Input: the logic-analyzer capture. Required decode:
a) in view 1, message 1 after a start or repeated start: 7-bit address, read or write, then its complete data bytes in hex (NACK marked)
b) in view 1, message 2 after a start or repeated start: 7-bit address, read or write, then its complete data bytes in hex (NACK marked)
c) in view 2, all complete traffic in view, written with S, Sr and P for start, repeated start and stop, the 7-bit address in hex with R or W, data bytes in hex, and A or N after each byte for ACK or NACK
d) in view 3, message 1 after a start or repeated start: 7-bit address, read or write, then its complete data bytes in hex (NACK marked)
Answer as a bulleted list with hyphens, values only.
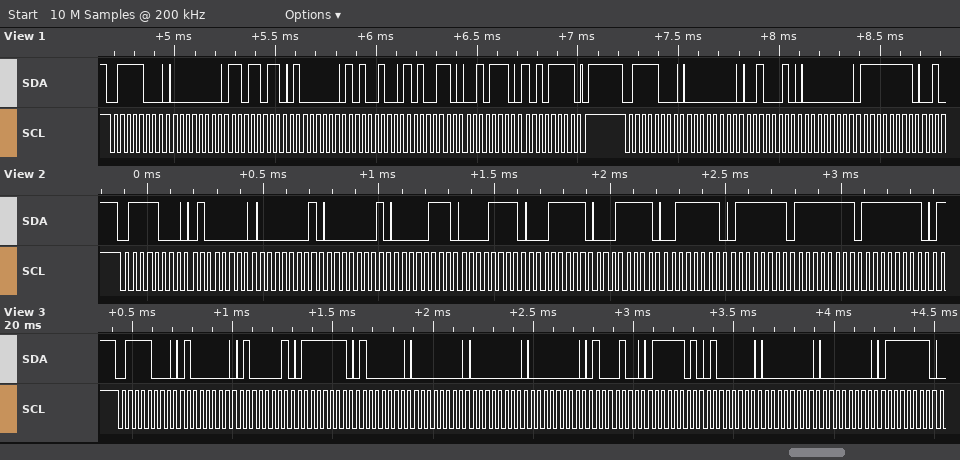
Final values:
- 0x3C write: 00 DB 40 A4 A6 2E AF
- 0x3C write: 00 22 00 FF
- S 3CW A 40 A 01 A 01 A 07 A 0F A 1F A 1F A 3F A 7F A FF A FF A
- 0x3C write: 40 41 7F 40 00 00 00 44 7D 40 00 00 7F
